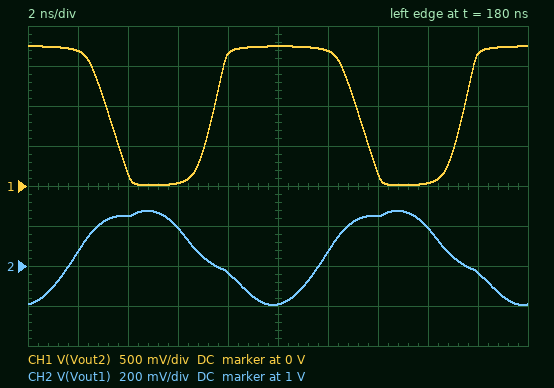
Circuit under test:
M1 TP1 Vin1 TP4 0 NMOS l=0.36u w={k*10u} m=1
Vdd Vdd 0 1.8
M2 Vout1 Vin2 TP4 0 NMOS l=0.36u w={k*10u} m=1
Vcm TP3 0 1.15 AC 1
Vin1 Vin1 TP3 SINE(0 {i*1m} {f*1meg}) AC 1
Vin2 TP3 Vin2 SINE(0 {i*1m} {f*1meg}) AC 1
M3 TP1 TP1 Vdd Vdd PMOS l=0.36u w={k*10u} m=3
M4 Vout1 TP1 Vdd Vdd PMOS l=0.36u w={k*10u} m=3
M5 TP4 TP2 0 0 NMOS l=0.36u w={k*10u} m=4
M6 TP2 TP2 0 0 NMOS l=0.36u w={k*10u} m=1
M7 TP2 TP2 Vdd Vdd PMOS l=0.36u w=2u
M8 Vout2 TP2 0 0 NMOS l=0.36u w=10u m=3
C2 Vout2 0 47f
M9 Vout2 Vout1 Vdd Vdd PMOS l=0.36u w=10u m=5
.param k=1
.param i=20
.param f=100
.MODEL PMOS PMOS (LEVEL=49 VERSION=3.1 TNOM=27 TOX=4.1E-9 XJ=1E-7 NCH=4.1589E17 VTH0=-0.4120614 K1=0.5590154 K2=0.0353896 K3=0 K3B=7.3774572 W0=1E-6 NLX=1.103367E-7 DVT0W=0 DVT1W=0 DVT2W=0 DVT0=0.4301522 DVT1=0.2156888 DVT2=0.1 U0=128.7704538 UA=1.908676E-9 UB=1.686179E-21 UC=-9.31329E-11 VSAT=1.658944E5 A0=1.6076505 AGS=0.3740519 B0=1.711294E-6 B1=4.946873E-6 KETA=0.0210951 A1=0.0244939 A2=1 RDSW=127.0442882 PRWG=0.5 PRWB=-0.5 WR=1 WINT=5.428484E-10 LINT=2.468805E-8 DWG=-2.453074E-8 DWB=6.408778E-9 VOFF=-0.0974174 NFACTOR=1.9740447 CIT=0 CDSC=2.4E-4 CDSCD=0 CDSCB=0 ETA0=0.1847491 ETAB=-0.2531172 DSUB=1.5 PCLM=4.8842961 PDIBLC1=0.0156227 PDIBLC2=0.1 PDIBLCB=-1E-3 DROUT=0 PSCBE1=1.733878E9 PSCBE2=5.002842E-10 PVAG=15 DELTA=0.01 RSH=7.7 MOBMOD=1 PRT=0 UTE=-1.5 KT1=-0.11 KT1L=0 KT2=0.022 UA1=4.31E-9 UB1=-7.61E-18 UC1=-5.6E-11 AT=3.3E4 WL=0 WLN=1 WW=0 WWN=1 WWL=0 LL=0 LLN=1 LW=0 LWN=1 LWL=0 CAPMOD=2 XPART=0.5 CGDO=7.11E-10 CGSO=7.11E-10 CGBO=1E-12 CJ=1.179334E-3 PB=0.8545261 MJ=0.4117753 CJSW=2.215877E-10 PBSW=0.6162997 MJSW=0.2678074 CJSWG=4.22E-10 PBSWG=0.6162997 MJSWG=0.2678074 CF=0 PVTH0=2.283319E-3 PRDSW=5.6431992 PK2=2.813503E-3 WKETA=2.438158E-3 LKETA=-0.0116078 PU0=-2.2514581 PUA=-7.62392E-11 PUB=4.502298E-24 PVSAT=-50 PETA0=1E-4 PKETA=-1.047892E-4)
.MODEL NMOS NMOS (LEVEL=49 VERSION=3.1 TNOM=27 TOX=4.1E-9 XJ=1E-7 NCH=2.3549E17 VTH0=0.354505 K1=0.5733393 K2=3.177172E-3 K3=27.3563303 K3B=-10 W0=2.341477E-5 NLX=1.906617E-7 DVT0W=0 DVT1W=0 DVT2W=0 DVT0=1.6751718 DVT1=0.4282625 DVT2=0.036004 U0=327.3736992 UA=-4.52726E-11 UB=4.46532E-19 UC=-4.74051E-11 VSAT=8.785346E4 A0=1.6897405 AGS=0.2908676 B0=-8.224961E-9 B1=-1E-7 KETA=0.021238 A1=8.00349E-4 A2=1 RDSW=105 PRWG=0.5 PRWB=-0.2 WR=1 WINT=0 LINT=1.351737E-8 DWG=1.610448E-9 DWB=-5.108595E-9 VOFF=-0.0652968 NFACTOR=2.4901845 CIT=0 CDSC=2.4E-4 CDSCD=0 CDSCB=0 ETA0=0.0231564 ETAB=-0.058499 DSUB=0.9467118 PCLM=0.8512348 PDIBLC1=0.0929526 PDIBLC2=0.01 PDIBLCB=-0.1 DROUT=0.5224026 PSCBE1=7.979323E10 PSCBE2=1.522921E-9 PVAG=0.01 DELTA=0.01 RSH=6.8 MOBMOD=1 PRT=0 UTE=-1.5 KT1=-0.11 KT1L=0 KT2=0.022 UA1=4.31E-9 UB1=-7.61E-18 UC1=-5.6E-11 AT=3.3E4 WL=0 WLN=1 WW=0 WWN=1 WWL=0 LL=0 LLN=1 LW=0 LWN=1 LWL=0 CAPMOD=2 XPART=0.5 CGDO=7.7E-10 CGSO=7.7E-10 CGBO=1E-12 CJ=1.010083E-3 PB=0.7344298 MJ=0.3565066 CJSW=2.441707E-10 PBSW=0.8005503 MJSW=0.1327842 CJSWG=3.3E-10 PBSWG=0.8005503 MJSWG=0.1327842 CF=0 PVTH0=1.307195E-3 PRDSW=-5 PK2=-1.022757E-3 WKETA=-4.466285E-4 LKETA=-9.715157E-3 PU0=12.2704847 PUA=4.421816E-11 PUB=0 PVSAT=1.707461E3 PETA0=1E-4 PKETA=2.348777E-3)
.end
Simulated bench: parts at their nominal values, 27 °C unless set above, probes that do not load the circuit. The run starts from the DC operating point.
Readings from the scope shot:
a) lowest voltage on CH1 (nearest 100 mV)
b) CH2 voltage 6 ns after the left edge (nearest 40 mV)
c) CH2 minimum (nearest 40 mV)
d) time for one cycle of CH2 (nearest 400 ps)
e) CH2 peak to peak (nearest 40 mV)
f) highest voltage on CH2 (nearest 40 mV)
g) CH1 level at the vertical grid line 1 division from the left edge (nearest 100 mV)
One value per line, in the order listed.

0 V
1.20 V
800 mV
10.0 ns
480 mV
1.28 V
1.7 V
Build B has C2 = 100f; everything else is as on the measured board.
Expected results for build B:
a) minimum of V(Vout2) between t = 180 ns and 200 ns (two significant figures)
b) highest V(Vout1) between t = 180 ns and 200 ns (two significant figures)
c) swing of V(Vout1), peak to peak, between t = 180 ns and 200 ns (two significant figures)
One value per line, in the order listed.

9.5 mV
1.3 V
480 mV
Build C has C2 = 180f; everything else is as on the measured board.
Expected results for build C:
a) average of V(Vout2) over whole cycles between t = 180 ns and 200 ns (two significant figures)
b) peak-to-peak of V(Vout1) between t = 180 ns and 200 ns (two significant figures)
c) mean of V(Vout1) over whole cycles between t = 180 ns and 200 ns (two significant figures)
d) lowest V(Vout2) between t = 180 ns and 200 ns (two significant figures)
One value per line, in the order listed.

1.1 V
520 mV
1.1 V
10 mV
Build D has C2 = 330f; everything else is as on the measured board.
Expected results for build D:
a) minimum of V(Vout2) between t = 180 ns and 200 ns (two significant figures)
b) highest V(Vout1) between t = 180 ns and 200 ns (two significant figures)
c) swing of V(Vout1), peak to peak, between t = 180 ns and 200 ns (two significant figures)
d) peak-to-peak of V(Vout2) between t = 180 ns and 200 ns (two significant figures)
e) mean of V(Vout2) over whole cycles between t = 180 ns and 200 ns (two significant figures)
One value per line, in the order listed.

51 mV
1.4 V
580 mV
1.7 V
1.1 V
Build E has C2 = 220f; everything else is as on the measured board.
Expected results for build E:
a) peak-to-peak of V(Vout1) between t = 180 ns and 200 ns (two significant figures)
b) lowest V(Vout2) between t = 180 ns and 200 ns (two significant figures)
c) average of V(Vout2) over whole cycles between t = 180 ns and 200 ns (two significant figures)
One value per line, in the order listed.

540 mV
14 mV
1.1 V
